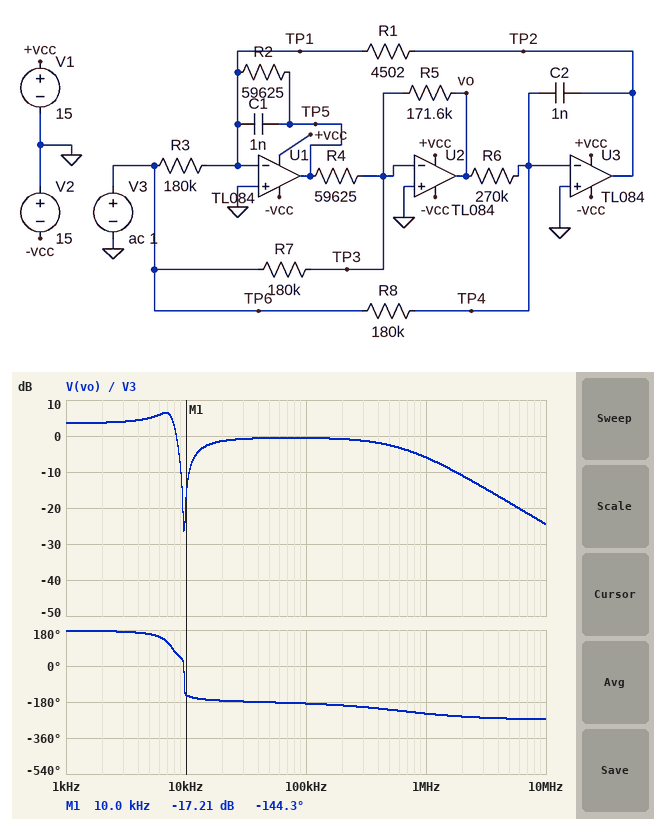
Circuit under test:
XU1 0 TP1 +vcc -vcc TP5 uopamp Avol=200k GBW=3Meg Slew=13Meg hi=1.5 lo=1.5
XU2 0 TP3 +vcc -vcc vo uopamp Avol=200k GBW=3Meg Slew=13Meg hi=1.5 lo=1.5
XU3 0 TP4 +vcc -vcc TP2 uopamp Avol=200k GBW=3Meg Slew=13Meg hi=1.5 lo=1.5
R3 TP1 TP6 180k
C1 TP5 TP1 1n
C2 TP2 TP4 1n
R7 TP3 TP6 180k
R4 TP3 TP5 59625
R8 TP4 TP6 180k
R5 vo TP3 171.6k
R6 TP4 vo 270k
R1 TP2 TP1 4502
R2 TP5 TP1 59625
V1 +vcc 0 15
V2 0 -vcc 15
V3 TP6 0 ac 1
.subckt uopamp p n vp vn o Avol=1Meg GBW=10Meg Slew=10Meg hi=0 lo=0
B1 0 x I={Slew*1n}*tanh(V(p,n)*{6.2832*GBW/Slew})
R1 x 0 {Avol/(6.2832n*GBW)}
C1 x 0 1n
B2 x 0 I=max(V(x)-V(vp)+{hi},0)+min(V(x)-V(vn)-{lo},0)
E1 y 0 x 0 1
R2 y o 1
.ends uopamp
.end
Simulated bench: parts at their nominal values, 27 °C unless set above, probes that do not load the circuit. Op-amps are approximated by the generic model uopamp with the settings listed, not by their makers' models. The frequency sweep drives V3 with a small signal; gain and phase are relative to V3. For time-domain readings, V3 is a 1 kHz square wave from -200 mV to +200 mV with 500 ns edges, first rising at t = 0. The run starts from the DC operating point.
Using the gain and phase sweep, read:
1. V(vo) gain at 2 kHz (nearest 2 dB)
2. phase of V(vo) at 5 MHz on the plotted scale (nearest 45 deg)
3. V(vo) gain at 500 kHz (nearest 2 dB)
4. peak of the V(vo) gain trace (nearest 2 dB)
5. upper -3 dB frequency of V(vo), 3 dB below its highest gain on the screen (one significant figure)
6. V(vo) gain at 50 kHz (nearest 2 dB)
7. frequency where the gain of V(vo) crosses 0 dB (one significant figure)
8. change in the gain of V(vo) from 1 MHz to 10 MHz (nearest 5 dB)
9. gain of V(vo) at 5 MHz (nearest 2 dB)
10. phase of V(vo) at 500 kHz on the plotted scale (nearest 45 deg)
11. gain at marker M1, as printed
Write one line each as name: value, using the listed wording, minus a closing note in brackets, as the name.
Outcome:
V(vo) gain at 2 kHz: 4 dB
phase of V(vo) at 5 MHz on the plotted scale: -270 deg
V(vo) gain at 500 kHz: -2 dB
peak of the V(vo) gain trace: 6 dB
upper -3 dB frequency of V(vo), 3 dB below its highest gain on the screen: 8 kHz
V(vo) gain at 50 kHz: 0 dB
frequency where the gain of V(vo) crosses 0 dB: 8 kHz
change in the gain of V(vo) from 1 MHz to 10 MHz: -20 dB
gain of V(vo) at 5 MHz: -18 dB
phase of V(vo) at 500 kHz on the plotted scale: -225 deg
gain at marker M1, as printed: -17.21 dB
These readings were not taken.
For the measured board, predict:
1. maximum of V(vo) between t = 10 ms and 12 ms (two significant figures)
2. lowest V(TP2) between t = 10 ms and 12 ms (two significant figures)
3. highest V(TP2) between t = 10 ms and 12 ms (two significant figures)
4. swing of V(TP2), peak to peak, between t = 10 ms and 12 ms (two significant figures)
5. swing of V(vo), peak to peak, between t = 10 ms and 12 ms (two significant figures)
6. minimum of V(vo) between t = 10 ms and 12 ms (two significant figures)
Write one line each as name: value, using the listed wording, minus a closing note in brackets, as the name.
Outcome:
maximum of V(vo) between t = 10 ms and 12 ms: 450 mV
lowest V(TP2) between t = 10 ms and 12 ms: -22 mV
highest V(TP2) between t = 10 ms and 12 ms: 22 mV
swing of V(TP2), peak to peak, between t = 10 ms and 12 ms: 44 mV
swing of V(vo), peak to peak, between t = 10 ms and 12 ms: 900 mV
minimum of V(vo) between t = 10 ms and 12 ms: -450 mV
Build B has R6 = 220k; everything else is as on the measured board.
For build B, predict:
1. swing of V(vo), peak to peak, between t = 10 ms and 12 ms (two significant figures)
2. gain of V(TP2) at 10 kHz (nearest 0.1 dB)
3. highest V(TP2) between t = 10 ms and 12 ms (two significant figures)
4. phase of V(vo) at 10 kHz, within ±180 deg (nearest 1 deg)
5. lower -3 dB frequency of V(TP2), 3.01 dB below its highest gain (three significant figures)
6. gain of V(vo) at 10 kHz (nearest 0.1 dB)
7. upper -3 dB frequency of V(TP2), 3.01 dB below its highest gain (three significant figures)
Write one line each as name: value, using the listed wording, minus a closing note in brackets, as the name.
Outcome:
swing of V(vo), peak to peak, between t = 10 ms and 12 ms: 680 mV
gain of V(TP2) at 10 kHz: -21.9 dB
highest V(TP2) between t = 10 ms and 12 ms: 16 mV
phase of V(vo) at 10 kHz, within ±180 deg: -134 deg
lower -3 dB frequency of V(TP2), 3.01 dB below its highest gain: 7.11 kHz
gain of V(vo) at 10 kHz: -14.9 dB
upper -3 dB frequency of V(TP2), 3.01 dB below its highest gain: 9.61 kHz
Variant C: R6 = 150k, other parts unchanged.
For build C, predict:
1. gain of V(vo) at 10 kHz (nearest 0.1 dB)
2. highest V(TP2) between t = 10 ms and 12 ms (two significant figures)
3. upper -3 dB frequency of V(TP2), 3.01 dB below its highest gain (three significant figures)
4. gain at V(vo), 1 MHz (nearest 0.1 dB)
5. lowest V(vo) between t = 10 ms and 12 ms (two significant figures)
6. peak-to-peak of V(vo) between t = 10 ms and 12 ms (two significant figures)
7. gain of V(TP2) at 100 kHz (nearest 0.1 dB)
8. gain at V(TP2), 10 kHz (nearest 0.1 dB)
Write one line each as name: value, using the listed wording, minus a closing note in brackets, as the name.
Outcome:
gain of V(vo) at 10 kHz: -11.5 dB
highest V(TP2) between t = 10 ms and 12 ms: 11 mV
upper -3 dB frequency of V(TP2), 3.01 dB below its highest gain: 11.4 kHz
gain at V(vo), 1 MHz: -6.0 dB
lowest V(vo) between t = 10 ms and 12 ms: -220 mV
peak-to-peak of V(vo) between t = 10 ms and 12 ms: 440 mV
gain of V(TP2) at 100 kHz: -55.3 dB
gain at V(TP2), 10 kHz: -19.9 dB
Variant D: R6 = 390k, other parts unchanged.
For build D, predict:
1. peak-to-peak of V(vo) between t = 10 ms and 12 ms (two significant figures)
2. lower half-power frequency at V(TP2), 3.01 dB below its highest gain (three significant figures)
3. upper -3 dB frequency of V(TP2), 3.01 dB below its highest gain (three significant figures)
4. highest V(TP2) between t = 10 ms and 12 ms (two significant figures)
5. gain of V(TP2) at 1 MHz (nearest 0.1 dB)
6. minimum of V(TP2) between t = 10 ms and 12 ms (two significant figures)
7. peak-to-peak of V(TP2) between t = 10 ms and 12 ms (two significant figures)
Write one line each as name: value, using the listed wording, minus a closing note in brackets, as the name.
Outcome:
peak-to-peak of V(vo) between t = 10 ms and 12 ms: 1.4 V
lower half-power frequency at V(TP2), 3.01 dB below its highest gain: 5.07 kHz
upper -3 dB frequency of V(TP2), 3.01 dB below its highest gain: 7.63 kHz
highest V(TP2) between t = 10 ms and 12 ms: 34 mV
gain of V(TP2) at 1 MHz: -62.4 dB
minimum of V(TP2) between t = 10 ms and 12 ms: -34 mV
peak-to-peak of V(TP2) between t = 10 ms and 12 ms: 67 mV
